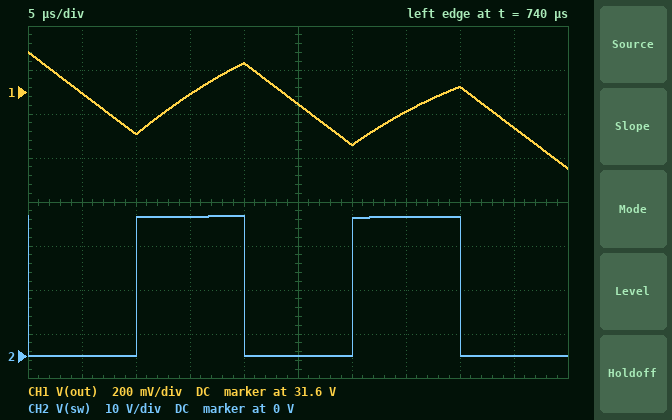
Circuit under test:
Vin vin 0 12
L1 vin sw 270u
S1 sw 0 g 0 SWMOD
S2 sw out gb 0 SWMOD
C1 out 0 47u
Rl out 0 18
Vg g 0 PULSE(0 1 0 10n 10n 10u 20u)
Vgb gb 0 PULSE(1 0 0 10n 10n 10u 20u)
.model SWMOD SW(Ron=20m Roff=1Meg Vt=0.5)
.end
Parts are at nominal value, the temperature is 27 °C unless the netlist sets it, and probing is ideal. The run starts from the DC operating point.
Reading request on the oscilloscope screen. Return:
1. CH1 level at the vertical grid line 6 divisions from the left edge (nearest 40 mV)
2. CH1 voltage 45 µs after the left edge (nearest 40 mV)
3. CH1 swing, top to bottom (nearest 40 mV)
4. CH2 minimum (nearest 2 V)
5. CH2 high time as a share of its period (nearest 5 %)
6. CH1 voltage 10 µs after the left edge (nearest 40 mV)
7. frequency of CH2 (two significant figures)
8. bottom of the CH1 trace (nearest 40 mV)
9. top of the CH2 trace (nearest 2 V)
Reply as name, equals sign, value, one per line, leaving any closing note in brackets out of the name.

CH1 level at the vertical grid line 6 divisions from the left edge = 31.36 V
CH1 voltage 45 µs after the left edge = 31.44 V
CH1 swing, top to bottom = 520 mV
CH2 minimum = 0 V
CH2 high time as a share of its period = 50 %
CH1 voltage 10 µs after the left edge = 31.40 V
frequency of CH2 = 50 kHz
bottom of the CH1 trace = 31.24 V
top of the CH2 trace = 32 V
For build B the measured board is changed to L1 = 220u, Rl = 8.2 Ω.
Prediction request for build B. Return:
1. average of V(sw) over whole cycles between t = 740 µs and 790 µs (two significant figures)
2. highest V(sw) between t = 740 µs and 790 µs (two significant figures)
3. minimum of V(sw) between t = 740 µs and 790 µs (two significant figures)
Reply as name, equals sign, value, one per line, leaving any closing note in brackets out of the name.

average of V(sw) over whole cycles between t = 740 µs and 790 µs = 14 V
highest V(sw) between t = 740 µs and 790 µs = 29 V
minimum of V(sw) between t = 740 µs and 790 µs = 120 mV
